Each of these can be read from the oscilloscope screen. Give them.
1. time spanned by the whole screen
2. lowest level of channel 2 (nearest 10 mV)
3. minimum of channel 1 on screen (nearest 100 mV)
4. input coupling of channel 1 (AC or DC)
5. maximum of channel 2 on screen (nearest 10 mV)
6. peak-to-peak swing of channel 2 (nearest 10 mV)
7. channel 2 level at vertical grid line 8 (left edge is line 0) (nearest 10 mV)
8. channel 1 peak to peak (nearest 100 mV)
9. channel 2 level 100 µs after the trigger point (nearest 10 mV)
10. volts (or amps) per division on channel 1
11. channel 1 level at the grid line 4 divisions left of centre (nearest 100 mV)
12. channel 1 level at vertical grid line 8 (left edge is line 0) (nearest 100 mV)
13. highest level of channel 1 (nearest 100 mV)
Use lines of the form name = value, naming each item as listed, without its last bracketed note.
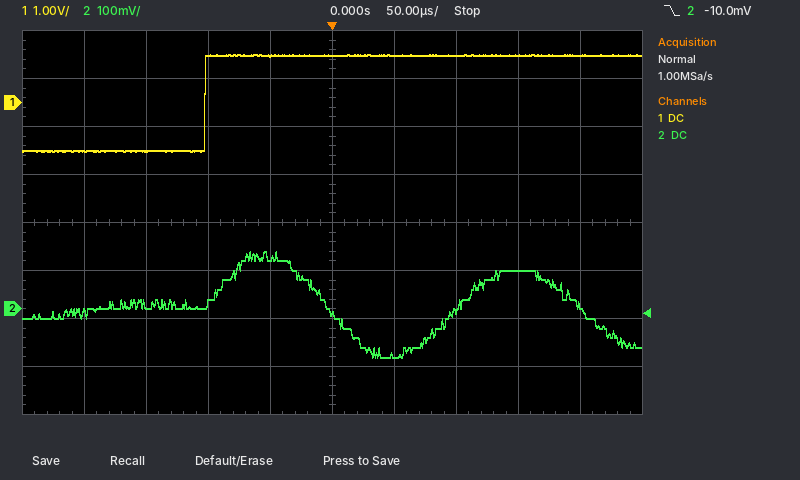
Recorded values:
time spanned by the whole screen = 500 µs
lowest level of channel 2 = -100 mV
minimum of channel 1 on screen = -1.0 V
input coupling of channel 1 = DC
maximum of channel 2 on screen = 120 mV
peak-to-peak swing of channel 2 = 220 mV
channel 2 level at vertical grid line 8 (left edge is line 0) = 80 mV
channel 1 peak to peak = 2.0 V
channel 2 level 100 µs after the trigger point = 0 mV
volts (or amps) per division on channel 1 = 1 V
channel 1 level at the grid line 4 divisions left of centre = -1.0 V
channel 1 level at vertical grid line 8 (left edge is line 0) = 1.0 V
highest level of channel 1 = 1.0 V
